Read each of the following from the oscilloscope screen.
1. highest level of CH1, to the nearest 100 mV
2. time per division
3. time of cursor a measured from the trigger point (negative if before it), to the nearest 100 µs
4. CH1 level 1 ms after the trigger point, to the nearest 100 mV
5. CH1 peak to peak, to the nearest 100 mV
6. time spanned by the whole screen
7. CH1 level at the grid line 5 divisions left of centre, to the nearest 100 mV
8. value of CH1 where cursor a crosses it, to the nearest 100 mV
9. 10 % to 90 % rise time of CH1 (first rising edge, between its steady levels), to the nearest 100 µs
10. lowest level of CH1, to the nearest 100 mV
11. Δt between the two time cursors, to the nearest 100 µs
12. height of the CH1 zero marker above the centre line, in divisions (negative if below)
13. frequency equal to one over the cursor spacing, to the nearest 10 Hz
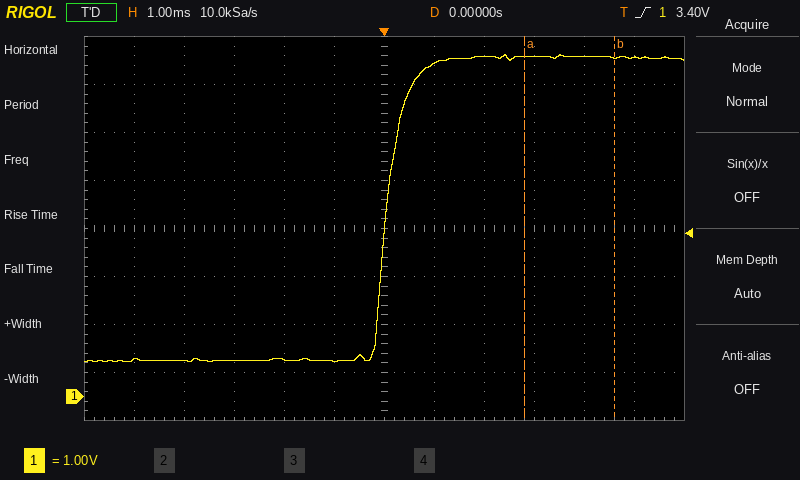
7.1 V
1 ms
+2.8 ms
6.9 V
6.4 V
12 ms
800 mV
7.1 V
700 µs
700 mV
1.8 ms
-3.5 div
560 Hz
